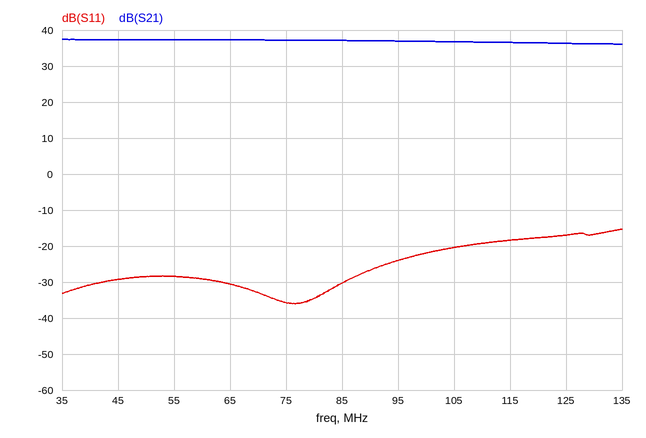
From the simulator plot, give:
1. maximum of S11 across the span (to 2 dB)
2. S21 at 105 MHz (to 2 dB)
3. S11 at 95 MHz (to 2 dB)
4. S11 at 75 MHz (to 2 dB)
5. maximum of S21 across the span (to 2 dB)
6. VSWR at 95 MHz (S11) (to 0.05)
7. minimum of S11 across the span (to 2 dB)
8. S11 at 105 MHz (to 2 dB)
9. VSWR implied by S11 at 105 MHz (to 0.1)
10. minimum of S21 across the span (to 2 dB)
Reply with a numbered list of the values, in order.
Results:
1. -16 dB
2. 36 dB
3. -24 dB
4. -36 dB
5. 38 dB
6. 1.15
7. -36 dB
8. -20 dB
9. 1.2
10. 36 dB
